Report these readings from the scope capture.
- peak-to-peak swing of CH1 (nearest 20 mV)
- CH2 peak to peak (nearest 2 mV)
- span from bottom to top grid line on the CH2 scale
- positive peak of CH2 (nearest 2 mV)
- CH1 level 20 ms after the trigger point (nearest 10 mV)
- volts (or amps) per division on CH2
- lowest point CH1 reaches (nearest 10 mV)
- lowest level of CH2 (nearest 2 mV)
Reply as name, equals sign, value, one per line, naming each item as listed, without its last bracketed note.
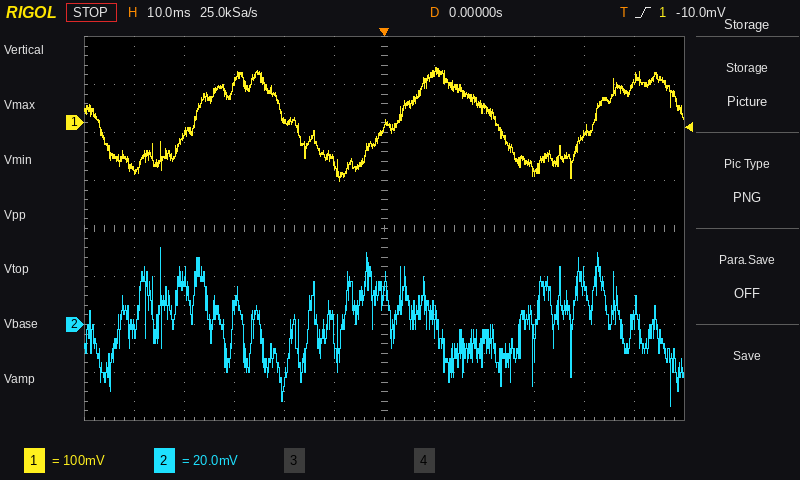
peak-to-peak swing of CH1 = 240 mV
CH2 peak to peak = 66 mV
span from bottom to top grid line on the CH2 scale = 160 mV
positive peak of CH2 = 32 mV
CH1 level 20 ms after the trigger point = 30 mV
volts (or amps) per division on CH2 = 20 mV
lowest point CH1 reaches = -120 mV
lowest level of CH2 = -34 mV
